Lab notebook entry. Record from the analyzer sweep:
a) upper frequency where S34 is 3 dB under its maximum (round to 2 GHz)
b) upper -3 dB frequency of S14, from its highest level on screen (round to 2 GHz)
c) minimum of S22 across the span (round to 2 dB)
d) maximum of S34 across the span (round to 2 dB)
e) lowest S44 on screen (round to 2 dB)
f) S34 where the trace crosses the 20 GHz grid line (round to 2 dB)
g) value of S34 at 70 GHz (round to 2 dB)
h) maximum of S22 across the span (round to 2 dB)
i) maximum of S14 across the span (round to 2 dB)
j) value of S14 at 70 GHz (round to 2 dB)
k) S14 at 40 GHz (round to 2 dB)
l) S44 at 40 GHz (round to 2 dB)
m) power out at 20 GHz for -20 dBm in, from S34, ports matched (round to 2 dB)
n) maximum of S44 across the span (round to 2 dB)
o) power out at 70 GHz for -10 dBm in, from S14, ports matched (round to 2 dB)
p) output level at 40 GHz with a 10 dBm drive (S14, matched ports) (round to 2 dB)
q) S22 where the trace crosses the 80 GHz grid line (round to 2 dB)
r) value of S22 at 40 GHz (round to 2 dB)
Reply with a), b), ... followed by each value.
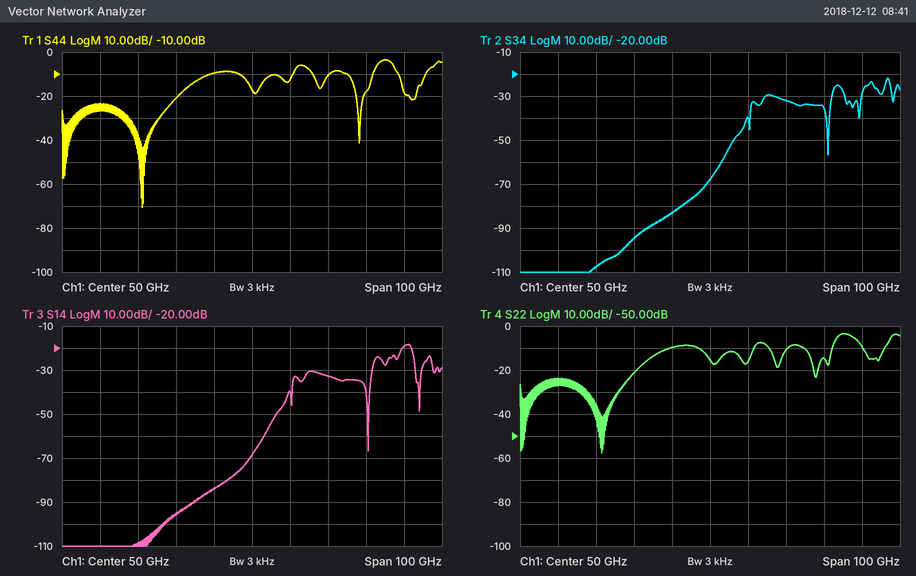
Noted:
a) 98 GHz
b) 92 GHz
c) -58 dB
d) -22 dB
e) -70 dB
f) -108 dB
g) -32 dB
h) -4 dB
i) -18 dB
j) -32 dB
k) -84 dB
l) -10 dB
m) -128 dBm
n) -4 dB
o) -42 dBm
p) -74 dBm
q) -14 dB
r) -10 dB
